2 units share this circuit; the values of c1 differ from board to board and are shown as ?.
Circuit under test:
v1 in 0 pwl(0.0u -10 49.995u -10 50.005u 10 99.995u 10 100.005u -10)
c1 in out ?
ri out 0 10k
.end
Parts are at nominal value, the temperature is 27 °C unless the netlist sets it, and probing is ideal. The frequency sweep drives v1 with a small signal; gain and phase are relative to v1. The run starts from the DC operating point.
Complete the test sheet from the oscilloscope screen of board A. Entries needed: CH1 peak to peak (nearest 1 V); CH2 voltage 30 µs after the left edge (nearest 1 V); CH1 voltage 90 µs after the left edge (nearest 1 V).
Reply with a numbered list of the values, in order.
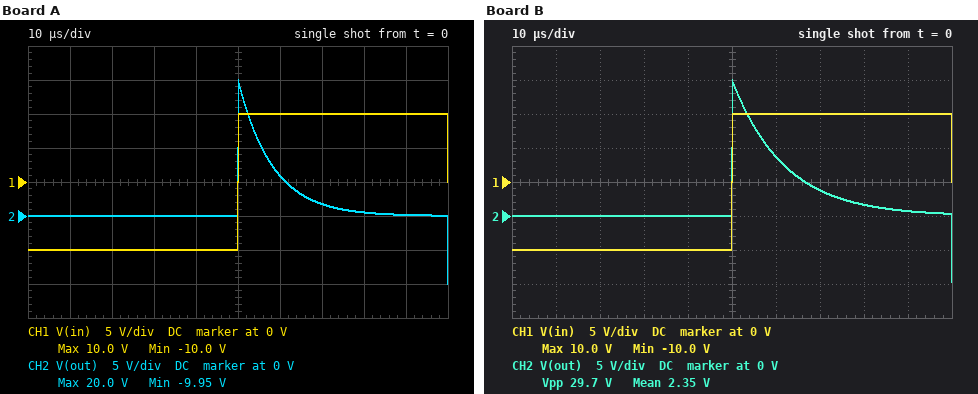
1. 20 V
2. 0 V
3. 10 V
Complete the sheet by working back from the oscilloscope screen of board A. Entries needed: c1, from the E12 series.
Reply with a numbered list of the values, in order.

1. 820 pF
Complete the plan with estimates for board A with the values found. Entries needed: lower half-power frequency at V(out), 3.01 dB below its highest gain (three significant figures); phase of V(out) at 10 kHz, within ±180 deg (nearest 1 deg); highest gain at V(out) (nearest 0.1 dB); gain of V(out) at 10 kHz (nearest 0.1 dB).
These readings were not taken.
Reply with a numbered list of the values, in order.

1. 19.4 kHz
2. 63 deg
3. 0 dB
4. -6.8 dB
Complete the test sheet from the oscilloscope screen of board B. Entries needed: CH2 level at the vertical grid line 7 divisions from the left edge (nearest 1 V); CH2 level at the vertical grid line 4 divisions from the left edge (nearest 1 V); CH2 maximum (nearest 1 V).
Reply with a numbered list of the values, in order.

1. 4 V
2. 0 V
3. 20 V
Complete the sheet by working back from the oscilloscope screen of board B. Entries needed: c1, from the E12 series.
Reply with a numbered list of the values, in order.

1. 1.2 nF
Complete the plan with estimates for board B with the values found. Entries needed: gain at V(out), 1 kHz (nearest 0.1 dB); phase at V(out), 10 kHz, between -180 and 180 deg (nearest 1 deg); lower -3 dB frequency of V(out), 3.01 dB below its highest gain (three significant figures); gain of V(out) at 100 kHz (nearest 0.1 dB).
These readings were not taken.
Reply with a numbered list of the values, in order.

1. -22.5 dB
2. 53 deg
3. 13.3 kHz
4. -0.1 dB
